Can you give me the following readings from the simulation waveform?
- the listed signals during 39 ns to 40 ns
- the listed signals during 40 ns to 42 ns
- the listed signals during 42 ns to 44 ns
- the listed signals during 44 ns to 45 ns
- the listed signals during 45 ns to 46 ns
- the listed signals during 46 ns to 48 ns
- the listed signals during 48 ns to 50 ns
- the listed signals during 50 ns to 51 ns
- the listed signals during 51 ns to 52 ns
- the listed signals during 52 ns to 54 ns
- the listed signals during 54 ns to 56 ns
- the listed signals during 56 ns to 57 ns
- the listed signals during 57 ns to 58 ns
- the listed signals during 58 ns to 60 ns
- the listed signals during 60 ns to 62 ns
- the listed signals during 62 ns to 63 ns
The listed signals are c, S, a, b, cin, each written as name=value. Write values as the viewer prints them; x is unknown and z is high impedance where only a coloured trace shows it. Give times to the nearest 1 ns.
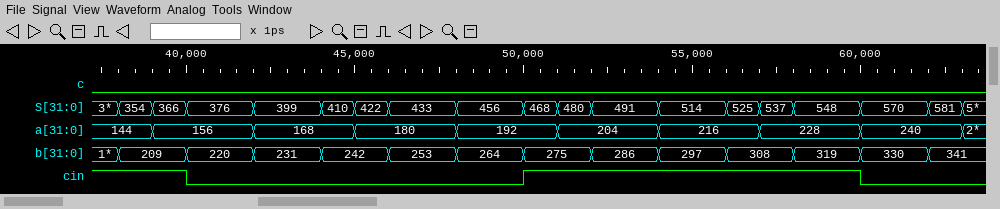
c=0, S=366, a=156, b=209, cin=1
c=0, S=376, a=156, b=220, cin=0
c=0, S=399, a=168, b=231, cin=0
c=0, S=410, a=168, b=242, cin=0
c=0, S=422, a=180, b=242, cin=0
c=0, S=433, a=180, b=253, cin=0
c=0, S=456, a=192, b=264, cin=0
c=0, S=468, a=192, b=275, cin=1
c=0, S=480, a=204, b=275, cin=1
c=0, S=491, a=204, b=286, cin=1
c=0, S=514, a=216, b=297, cin=1
c=0, S=525, a=216, b=308, cin=1
c=0, S=537, a=228, b=308, cin=1
c=0, S=548, a=228, b=319, cin=1
c=0, S=570, a=240, b=330, cin=0
c=0, S=581, a=240, b=341, cin=0
